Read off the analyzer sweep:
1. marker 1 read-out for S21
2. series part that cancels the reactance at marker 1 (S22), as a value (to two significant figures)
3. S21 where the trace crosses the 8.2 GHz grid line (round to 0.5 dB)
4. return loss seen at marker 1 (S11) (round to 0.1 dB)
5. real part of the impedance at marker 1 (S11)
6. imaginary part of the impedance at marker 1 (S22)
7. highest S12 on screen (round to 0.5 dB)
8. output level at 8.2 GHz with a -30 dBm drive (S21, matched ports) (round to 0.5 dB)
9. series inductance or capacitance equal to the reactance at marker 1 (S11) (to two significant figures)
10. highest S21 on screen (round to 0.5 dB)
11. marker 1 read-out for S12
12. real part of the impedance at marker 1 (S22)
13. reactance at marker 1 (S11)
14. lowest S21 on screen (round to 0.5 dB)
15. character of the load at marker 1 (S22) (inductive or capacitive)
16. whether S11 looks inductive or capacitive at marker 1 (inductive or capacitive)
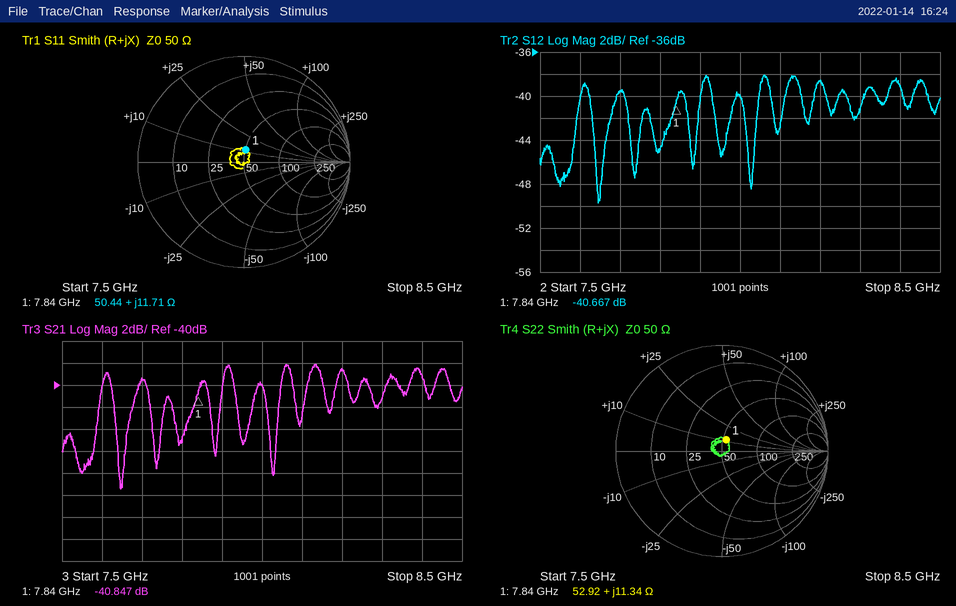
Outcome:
-40.847 dB
1.8 pF
-38.5 dB
18.7 dB
50.44 Ω
+11.34 Ω
-38.0 dB
-68.5 dBm
240 pH
-38.0 dB
-40.667 dB
52.92 Ω
+11.71 Ω
-49.5 dB
inductive
inductive
